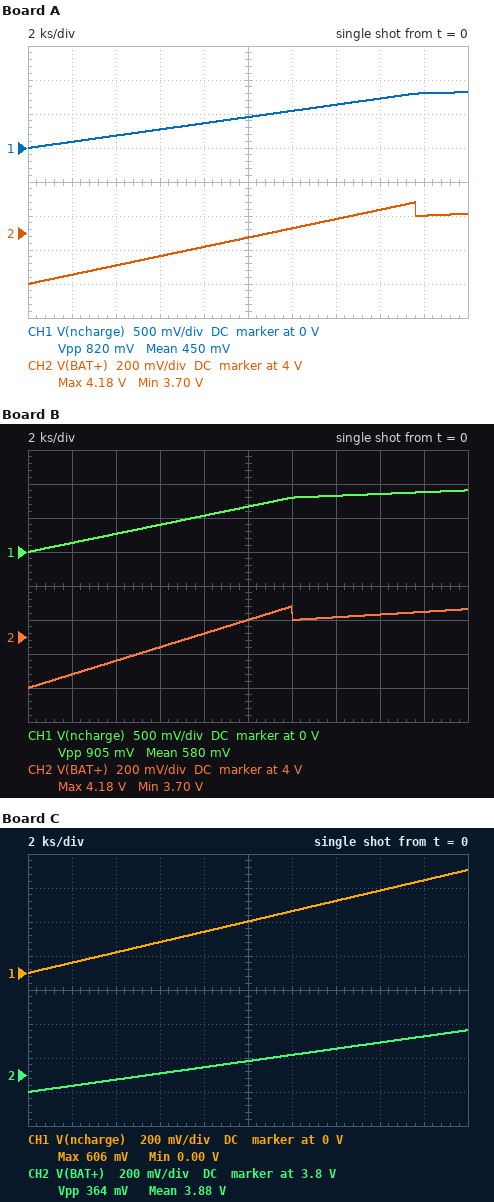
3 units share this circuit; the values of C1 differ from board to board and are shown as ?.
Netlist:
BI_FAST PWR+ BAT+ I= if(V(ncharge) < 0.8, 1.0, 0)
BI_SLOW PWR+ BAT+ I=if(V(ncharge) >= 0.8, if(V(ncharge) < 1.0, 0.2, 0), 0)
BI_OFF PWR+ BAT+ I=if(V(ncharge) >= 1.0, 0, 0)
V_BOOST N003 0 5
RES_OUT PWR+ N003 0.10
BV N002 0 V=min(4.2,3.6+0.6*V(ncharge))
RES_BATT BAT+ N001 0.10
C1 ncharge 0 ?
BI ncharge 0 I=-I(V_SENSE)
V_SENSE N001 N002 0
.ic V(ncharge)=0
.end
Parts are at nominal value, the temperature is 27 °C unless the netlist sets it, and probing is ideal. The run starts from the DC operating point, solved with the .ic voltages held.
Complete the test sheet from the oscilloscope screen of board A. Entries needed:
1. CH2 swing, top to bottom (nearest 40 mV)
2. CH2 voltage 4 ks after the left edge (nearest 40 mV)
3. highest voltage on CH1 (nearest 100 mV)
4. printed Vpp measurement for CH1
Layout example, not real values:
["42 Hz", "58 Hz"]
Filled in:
["480 mV", "3.80 V", "800 mV", "820 mV"]
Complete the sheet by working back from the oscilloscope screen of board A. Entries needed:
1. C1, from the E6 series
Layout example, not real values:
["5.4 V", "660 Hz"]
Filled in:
["22 kF"]
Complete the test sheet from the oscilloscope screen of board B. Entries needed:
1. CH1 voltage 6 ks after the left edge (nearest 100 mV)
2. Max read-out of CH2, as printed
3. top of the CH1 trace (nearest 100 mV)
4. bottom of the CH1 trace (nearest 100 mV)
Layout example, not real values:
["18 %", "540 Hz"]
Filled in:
["400 mV", "4.18 V", "900 mV", "0 V"]
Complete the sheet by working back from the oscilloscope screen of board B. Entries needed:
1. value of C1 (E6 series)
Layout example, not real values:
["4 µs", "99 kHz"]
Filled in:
["15 kF"]
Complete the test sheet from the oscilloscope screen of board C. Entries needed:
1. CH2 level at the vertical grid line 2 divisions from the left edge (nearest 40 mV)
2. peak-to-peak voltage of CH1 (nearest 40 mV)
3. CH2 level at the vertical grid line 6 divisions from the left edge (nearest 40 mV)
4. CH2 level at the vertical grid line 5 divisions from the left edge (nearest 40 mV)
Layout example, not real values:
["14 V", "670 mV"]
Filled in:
["3.76 V", "600 mV", "3.92 V", "3.88 V"]
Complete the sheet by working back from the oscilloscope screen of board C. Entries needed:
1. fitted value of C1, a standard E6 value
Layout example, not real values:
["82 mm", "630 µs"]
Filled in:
["33 kF"]
